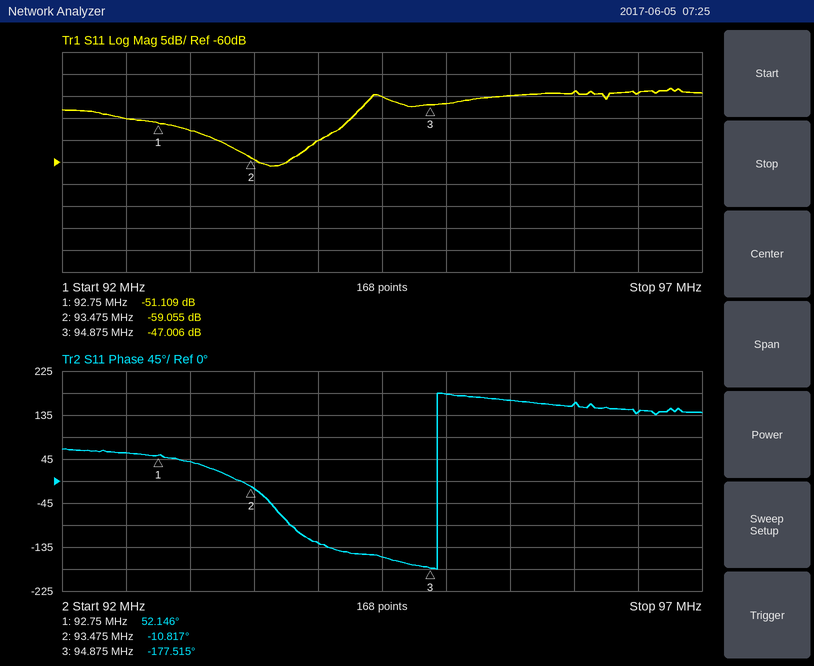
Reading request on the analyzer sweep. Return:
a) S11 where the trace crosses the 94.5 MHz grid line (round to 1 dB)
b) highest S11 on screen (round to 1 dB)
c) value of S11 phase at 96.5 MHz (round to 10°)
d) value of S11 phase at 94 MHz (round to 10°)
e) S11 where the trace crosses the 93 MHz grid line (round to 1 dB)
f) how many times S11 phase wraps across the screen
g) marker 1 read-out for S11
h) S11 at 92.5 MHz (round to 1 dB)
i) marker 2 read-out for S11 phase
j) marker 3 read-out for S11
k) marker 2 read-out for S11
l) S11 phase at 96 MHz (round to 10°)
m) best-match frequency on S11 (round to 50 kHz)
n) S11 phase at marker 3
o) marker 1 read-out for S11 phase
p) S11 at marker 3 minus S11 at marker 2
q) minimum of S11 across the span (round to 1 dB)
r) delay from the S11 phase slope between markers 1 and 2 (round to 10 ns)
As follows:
-45 dB
-43 dB
140°
-130°
-53 dB
1
-51.109 dB
-50 dB
-10.817°
-47.006 dB
-59.055 dB
160°
93.65 MHz
-177.515°
52.146°
12.049 dB
-61 dB
240 ns
